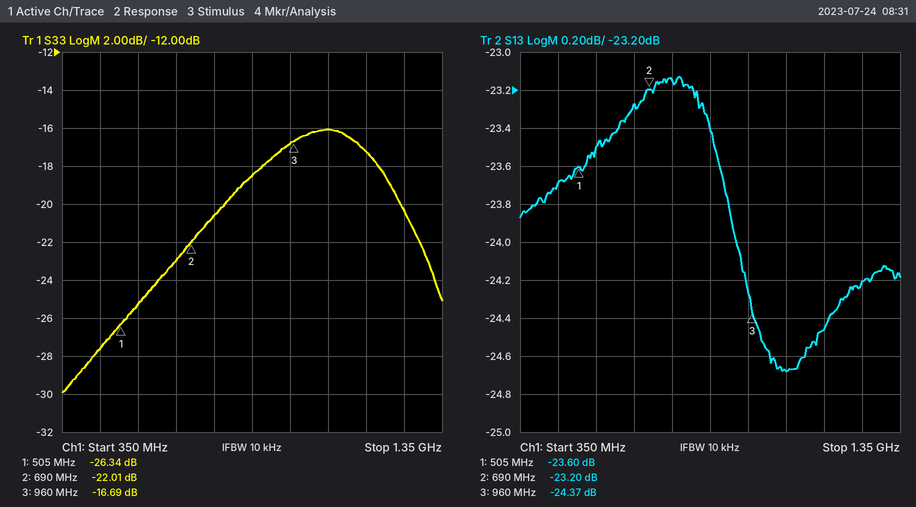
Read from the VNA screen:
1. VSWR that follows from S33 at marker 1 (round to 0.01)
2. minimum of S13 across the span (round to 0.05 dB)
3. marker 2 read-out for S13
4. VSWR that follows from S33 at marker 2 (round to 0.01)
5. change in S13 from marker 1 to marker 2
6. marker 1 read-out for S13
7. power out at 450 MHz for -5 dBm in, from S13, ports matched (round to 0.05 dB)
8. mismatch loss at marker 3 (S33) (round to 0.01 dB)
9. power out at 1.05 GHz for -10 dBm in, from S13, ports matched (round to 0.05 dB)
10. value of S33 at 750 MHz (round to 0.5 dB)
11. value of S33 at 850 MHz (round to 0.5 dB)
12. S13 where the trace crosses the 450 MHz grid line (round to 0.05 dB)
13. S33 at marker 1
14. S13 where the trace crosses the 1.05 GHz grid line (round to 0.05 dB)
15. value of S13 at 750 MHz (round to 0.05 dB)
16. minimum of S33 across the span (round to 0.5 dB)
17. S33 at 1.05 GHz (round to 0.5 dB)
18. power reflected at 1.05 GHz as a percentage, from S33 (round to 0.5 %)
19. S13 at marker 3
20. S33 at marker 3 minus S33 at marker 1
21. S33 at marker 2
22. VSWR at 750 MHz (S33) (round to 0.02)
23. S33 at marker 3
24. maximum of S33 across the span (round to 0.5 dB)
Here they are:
1.10
-24.70 dB
-23.20 dB
1.17
0.40 dB
-23.60 dB
-28.70 dBm
0.09 dB
-34.70 dBm
-20.5 dB
-18.5 dB
-23.70 dB
-26.34 dB
-24.70 dB
-23.15 dB
-30.0 dB
-16.0 dB
2.5 %
-24.37 dB
9.65 dB
-22.01 dB
1.20
-16.69 dB
-16.0 dB
